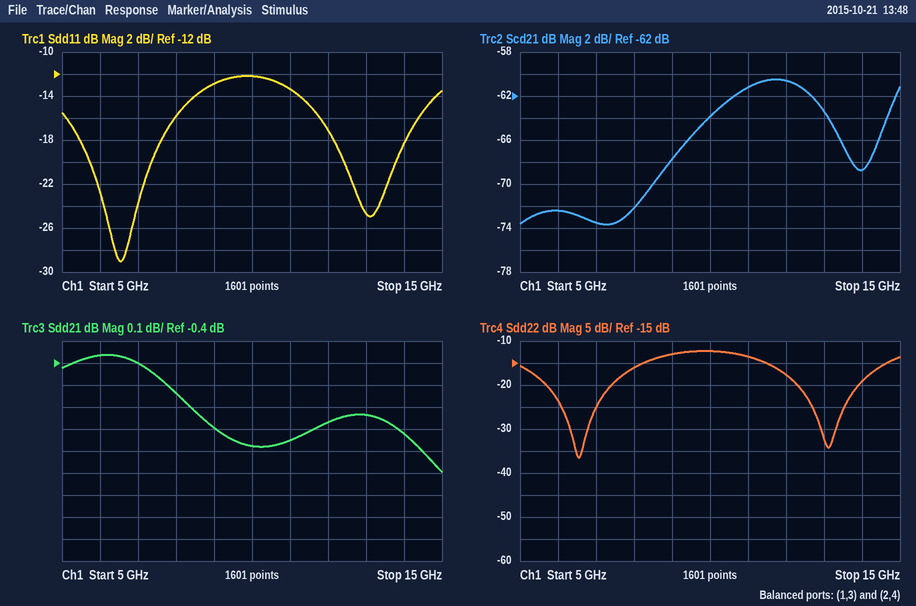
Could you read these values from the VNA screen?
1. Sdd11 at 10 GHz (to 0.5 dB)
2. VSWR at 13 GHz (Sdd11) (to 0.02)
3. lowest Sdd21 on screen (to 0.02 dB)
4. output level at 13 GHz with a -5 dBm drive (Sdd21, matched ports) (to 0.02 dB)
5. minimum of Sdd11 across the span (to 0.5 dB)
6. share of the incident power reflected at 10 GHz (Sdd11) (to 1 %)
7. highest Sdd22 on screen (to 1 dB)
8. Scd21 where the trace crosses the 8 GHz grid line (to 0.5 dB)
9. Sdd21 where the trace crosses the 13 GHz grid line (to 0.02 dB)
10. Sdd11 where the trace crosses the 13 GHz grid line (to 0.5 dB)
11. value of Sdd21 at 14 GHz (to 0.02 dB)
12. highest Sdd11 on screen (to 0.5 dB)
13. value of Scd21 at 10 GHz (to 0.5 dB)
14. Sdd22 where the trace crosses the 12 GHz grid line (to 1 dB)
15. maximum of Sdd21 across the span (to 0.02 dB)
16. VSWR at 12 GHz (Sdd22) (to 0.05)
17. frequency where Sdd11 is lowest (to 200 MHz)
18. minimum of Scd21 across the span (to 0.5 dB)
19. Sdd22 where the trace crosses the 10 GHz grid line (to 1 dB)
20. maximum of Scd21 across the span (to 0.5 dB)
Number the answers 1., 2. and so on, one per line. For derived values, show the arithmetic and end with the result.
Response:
1. -12.0 dB
2. |Γ| = 10^(-24.5/20) = 0.0596; VSWR = (1 + 0.0596)/(1 − 0.0596) ≈ 1.13, so 1.12 to the nearest 0.02
3. -0.90 dB
4. -5 dBm + (-0.64 dB) = -5.64 dBm
5. -29.0 dB
6. 10^(-12/10) ≈ 6 %
7. -12 dB
8. -72.0 dB
9. -0.64 dB
10. -24.5 dB
11. -0.72 dB
12. -12.0 dB
13. -64.0 dB
14. -18 dB
15. -0.36 dB
16. |Γ| = 10^(-18/20) = 0.1259; VSWR = (1 + 0.1259)/(1 − 0.1259) ≈ 1.29, so 1.30 to the nearest 0.05
17. 6.6 GHz
18. -73.5 dB
19. -12 dB
20. -60.5 dB
